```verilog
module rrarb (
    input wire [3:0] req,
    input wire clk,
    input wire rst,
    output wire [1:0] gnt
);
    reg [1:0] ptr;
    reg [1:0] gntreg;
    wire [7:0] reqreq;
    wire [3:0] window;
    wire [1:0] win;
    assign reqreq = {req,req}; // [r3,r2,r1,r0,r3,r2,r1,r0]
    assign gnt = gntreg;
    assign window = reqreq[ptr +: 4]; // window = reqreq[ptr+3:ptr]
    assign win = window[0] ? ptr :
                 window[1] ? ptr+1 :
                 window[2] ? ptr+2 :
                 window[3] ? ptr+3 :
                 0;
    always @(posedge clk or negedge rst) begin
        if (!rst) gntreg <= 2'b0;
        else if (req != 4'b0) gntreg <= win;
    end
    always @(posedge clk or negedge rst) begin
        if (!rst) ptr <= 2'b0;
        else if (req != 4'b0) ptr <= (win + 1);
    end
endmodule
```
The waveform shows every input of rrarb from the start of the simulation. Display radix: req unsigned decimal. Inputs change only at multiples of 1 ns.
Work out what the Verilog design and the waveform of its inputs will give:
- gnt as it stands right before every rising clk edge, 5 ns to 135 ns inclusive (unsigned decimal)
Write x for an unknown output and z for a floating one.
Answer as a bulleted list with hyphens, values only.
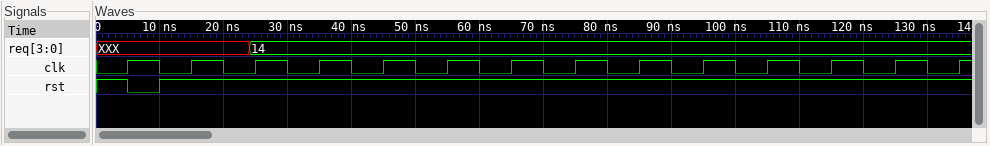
- x, 0, 0, 1, 2, 3, 1, 2, 3, 1, 2, 3, 1, 2
